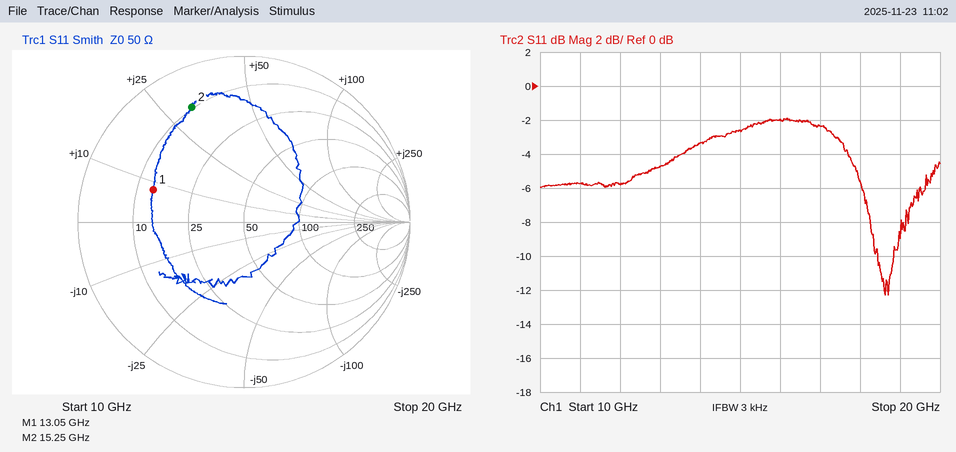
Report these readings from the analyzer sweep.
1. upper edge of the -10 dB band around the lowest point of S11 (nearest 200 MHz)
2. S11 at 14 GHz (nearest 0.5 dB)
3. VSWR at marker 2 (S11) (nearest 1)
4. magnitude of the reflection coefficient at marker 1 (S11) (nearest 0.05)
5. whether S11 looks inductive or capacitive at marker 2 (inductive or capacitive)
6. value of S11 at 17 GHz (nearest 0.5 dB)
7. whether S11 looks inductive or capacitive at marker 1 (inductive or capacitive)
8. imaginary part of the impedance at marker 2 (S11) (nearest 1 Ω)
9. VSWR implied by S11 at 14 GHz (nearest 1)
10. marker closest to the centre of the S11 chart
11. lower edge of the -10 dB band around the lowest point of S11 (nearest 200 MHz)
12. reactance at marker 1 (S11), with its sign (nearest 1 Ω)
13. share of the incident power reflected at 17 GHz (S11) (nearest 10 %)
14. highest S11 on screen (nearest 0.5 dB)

18.8 GHz
-3.5 dB
7
0.60
inductive
-2.5 dB
inductive
+31 Ω
5
marker 1
18.4 GHz
+8 Ω
60 %
-2.0 dB
